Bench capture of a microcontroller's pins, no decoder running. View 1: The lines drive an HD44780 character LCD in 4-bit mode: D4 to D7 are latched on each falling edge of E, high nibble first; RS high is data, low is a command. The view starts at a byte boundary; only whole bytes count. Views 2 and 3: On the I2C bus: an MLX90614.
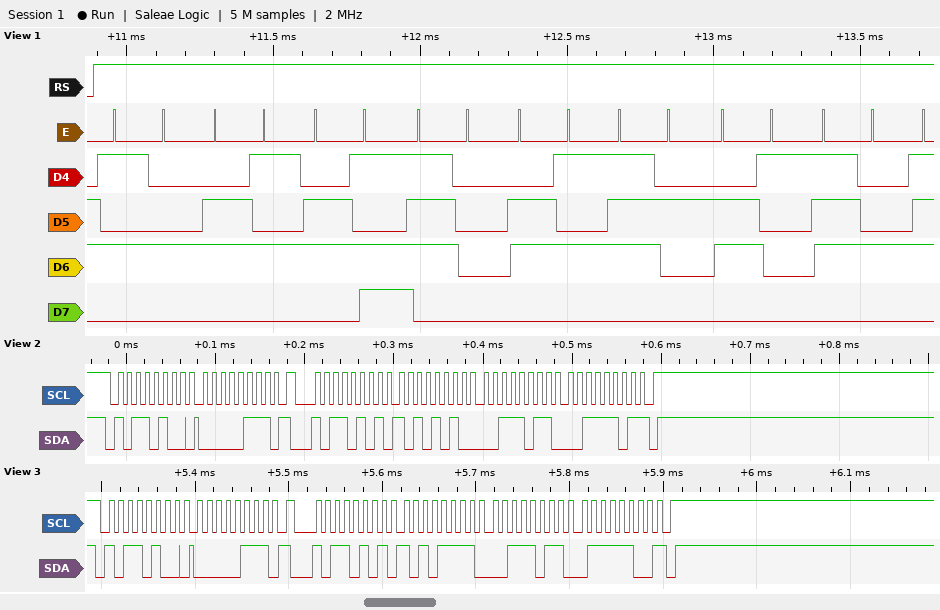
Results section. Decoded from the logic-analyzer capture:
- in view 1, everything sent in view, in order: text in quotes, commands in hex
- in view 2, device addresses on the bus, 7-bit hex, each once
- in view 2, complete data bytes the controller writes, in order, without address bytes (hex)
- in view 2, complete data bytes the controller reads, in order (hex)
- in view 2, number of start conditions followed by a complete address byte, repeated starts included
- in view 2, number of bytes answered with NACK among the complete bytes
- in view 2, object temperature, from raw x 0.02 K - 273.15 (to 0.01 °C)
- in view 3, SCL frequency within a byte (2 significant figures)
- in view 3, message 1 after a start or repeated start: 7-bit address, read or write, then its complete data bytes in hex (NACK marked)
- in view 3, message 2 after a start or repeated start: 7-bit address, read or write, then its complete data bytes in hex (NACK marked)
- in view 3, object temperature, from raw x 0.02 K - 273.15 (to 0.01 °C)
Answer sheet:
"Temperat"
0x5A
07
AA 3B 3D
2
1
32.33 °C
100 kHz
0x5A write: 07
0x5A read: AF 3B 7C NACK
32.43 °C
